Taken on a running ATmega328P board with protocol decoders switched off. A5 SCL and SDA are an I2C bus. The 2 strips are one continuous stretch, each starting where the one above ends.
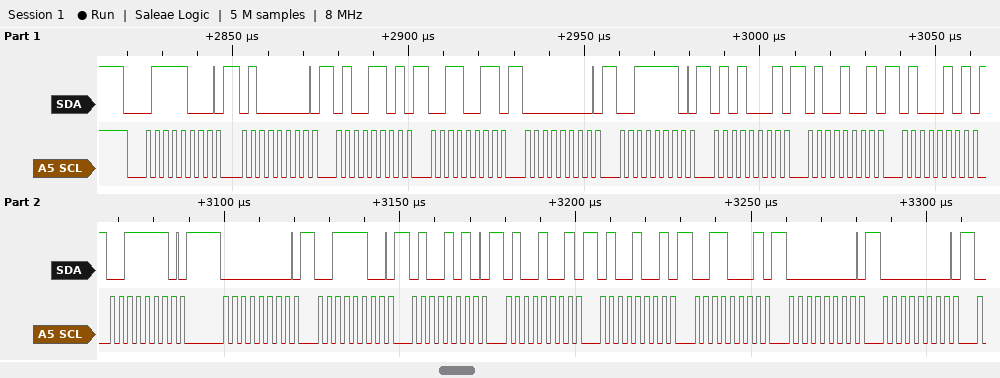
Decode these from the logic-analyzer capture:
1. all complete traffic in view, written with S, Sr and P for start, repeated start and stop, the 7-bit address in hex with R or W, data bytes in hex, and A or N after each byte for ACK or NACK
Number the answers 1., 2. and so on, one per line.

1. S 3CW A 40 A 4D A 33 A 00 A 3E A 51 A 49 A 45 A 3E A 00 A 3C A 4A A 49 A 49 A 31 A 00 A 00 A
